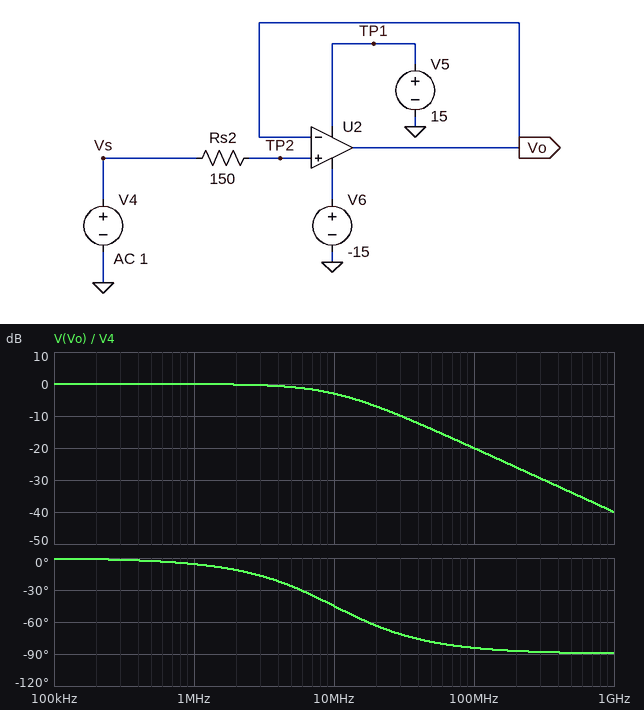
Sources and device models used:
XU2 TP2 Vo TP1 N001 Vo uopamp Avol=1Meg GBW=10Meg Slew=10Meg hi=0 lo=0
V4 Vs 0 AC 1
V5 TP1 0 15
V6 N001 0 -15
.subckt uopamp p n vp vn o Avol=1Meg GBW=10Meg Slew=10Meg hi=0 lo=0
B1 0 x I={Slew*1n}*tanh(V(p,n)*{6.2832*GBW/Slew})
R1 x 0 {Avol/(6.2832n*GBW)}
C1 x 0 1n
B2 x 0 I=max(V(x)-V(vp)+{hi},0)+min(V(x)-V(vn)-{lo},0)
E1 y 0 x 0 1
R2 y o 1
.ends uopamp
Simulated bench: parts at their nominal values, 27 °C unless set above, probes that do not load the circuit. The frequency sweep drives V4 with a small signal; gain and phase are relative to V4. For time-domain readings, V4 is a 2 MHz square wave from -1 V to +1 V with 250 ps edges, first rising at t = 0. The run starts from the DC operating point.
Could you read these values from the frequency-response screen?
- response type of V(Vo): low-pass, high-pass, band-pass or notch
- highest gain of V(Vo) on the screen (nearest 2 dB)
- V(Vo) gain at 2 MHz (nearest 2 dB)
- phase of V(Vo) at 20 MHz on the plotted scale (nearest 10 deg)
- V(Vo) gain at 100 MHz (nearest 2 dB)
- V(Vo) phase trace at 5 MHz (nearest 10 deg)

low-pass
0 dB
0 dB
-60 deg
-20 dB
-30 deg
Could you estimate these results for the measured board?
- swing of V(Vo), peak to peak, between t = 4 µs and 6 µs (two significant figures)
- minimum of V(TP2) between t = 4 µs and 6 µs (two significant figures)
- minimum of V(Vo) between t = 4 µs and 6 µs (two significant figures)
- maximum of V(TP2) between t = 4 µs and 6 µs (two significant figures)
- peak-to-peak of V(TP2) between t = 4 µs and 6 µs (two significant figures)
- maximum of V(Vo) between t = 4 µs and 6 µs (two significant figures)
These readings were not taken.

2.0 V
-1.0 V
-1.0 V
1.0 V
2.0 V
1.0 V
